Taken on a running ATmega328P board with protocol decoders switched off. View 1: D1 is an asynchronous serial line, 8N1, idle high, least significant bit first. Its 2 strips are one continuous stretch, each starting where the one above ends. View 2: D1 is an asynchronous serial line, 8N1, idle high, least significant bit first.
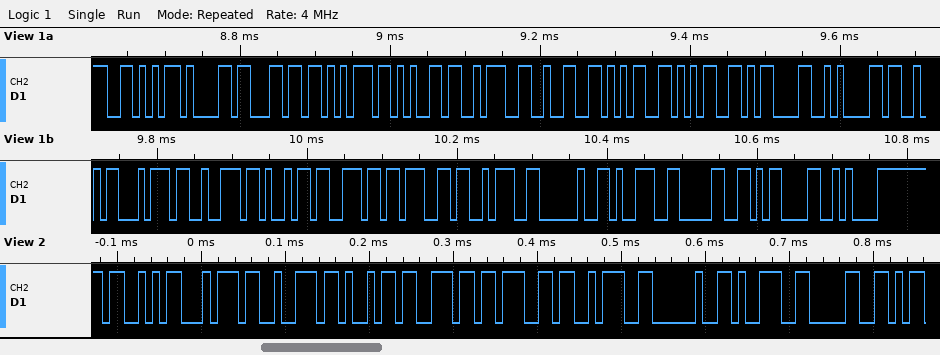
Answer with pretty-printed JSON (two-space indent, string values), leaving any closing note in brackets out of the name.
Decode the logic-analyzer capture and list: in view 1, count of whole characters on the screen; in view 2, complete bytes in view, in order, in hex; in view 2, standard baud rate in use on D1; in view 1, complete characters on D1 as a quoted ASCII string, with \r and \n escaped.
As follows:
{
  "in view 1, count of whole characters on the screen": "23",
  "in view 2, complete bytes in view, in order, in hex": "53 74 72 69 6E 67 3A 20 39 30",
  "in view 2, standard baud rate in use on D1": "115200 baud",
  "in view 1, complete characters on D1 as a quoted ASCII string, with \\r and \\n escaped": "\"Value:255\\r\\nString: 90\\r\\n\""
}
